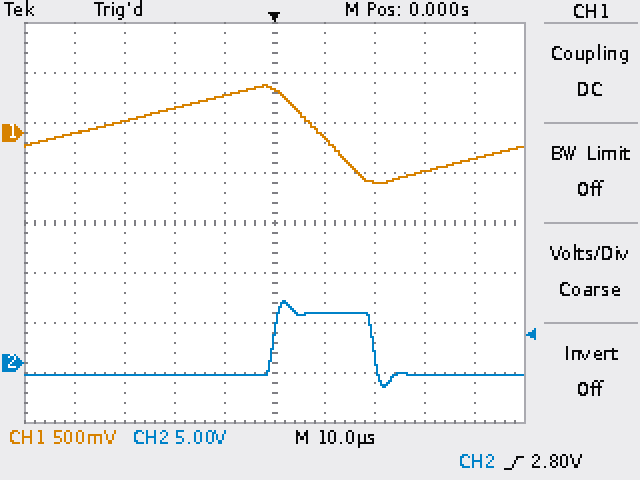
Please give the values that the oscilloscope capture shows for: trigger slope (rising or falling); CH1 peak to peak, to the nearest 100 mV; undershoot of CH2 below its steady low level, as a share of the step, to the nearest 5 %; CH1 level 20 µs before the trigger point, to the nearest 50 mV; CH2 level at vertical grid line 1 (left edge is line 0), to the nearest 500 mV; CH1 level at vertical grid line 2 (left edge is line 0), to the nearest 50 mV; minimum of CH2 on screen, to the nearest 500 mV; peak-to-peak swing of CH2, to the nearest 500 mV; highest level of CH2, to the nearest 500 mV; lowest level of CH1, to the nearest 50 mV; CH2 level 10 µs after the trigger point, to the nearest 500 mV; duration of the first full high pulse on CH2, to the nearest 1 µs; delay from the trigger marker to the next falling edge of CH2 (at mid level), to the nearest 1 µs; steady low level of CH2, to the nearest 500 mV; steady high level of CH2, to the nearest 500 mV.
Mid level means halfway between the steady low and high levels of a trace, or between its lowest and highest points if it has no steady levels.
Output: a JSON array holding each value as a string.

["rising", "1.00 V", "20 %", "250 mV", "-1.0 V", "100 mV", "-2.5 V", "8.5 V", "6.0 V", "-500 mV", "5.0 V", "20 µs", "20 µs", "-1.0 V", "5.0 V"]
